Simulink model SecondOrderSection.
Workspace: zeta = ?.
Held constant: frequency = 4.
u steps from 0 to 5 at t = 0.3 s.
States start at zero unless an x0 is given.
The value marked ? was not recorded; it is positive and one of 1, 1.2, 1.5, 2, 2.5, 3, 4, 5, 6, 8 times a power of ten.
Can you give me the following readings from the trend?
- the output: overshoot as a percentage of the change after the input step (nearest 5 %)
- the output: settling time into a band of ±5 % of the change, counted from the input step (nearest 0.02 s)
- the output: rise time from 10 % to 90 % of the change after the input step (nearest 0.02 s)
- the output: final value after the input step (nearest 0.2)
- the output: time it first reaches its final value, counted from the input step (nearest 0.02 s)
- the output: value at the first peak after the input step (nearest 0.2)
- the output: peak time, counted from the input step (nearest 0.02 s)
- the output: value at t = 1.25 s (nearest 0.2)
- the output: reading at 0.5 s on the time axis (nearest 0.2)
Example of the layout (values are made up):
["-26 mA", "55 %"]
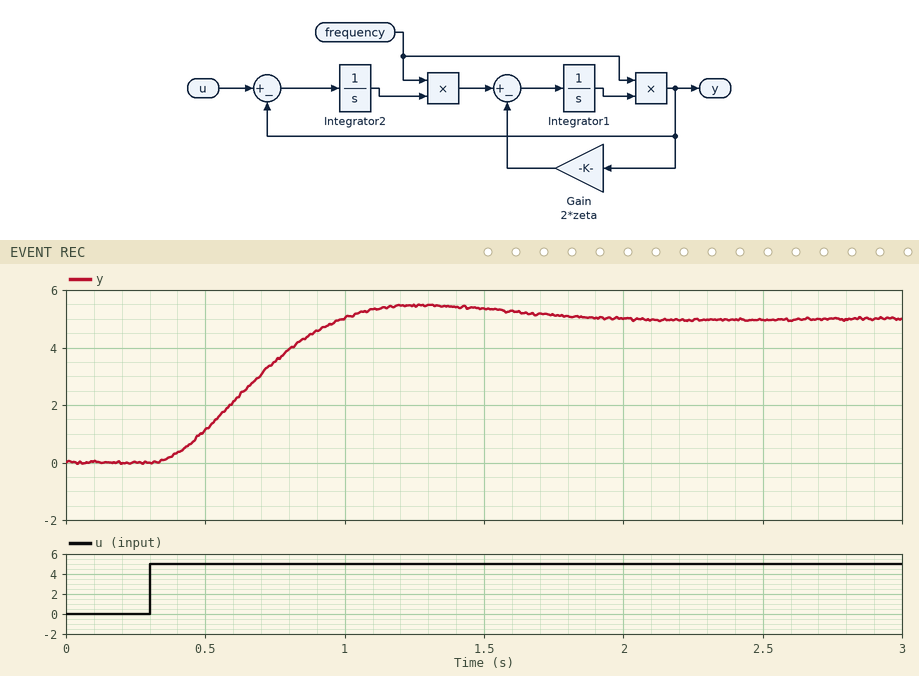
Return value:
["10 %", "1.30 s", "0.46 s", "5.0", "0.70 s", "5.4", "0.98 s", "5.4", "1.2"]
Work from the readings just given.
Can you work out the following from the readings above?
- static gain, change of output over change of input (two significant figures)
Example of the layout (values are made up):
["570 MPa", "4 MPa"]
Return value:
["1.0"]
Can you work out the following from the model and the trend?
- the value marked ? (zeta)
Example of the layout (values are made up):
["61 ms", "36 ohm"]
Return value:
["0.6"]
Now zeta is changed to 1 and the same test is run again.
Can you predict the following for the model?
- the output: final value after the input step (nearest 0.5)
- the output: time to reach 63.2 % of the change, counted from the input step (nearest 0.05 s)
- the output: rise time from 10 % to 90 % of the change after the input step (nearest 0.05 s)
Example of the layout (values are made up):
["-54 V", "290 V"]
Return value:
["5.0", "0.55 s", "0.85 s"]
